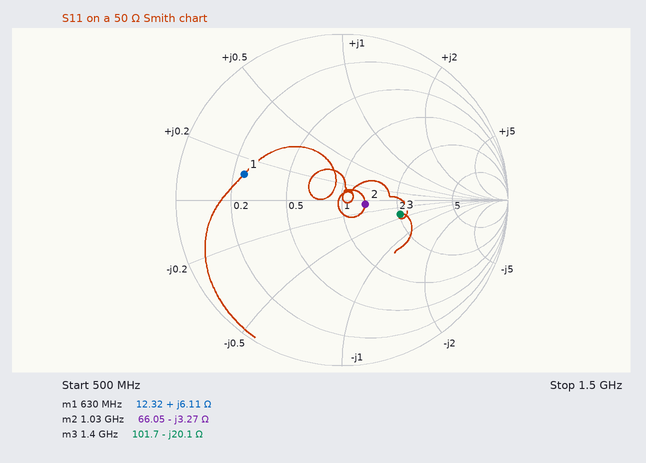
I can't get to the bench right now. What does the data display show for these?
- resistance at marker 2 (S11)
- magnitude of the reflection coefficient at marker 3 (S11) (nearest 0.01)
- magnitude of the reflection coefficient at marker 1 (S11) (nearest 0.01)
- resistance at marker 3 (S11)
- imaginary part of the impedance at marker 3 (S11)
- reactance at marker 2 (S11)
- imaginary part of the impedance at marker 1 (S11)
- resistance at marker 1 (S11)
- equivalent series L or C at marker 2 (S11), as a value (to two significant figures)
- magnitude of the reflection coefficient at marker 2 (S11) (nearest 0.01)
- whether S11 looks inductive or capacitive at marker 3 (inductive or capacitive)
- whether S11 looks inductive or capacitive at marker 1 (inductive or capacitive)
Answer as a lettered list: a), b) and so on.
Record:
a) 66.05 Ω
b) 0.36
c) 0.61
d) 101.7 Ω
e) -20.1 Ω
f) -3.27 Ω
g) +6.11 Ω
h) 12.32 Ω
i) 47 pF
j) 0.14
k) capacitive
l) inductive
